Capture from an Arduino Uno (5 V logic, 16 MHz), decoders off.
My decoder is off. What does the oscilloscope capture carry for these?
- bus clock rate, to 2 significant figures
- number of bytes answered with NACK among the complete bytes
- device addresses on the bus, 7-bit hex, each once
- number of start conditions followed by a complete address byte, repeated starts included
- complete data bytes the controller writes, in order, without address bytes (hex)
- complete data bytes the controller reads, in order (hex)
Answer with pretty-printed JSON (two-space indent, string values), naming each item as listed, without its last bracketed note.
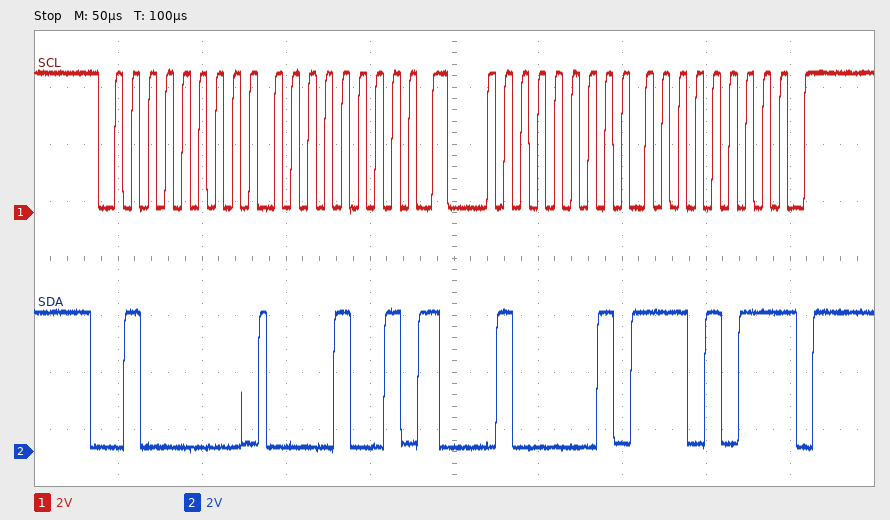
{
  "bus clock rate, to 2 significant figures": "100 kHz",
  "number of bytes answered with NACK among the complete bytes": "1",
  "device addresses on the bus, 7-bit hex, each once": "0x20",
  "number of start conditions followed by a complete address byte, repeated starts included": "2",
  "complete data bytes the controller writes, in order, without address bytes": "09",
  "complete data bytes the controller reads, in order": "EB"
}
